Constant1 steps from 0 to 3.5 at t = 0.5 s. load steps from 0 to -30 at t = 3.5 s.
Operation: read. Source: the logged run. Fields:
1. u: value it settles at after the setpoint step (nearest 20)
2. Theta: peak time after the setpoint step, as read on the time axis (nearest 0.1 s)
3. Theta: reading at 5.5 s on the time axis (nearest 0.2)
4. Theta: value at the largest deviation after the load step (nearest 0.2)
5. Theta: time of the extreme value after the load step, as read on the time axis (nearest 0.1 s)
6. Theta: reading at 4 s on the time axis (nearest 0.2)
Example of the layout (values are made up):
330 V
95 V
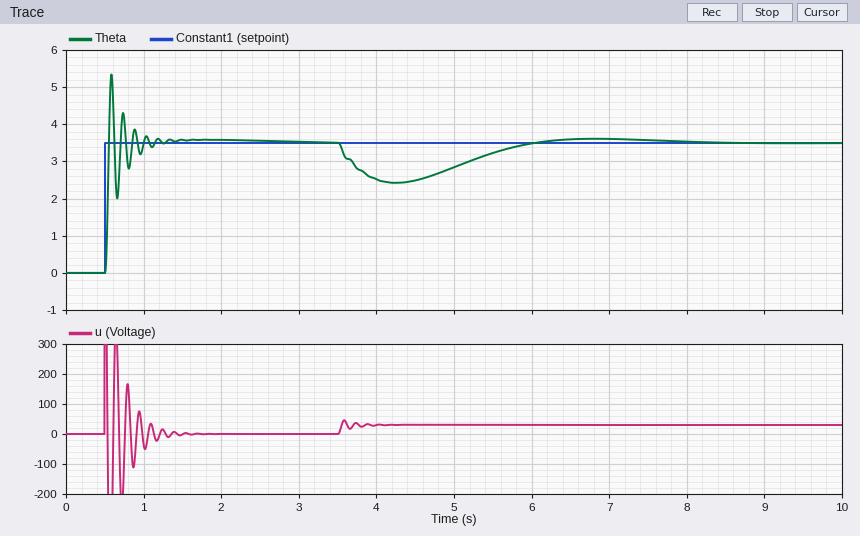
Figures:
0
0.6 s
3.2
2.4
4.2 s
2.6
